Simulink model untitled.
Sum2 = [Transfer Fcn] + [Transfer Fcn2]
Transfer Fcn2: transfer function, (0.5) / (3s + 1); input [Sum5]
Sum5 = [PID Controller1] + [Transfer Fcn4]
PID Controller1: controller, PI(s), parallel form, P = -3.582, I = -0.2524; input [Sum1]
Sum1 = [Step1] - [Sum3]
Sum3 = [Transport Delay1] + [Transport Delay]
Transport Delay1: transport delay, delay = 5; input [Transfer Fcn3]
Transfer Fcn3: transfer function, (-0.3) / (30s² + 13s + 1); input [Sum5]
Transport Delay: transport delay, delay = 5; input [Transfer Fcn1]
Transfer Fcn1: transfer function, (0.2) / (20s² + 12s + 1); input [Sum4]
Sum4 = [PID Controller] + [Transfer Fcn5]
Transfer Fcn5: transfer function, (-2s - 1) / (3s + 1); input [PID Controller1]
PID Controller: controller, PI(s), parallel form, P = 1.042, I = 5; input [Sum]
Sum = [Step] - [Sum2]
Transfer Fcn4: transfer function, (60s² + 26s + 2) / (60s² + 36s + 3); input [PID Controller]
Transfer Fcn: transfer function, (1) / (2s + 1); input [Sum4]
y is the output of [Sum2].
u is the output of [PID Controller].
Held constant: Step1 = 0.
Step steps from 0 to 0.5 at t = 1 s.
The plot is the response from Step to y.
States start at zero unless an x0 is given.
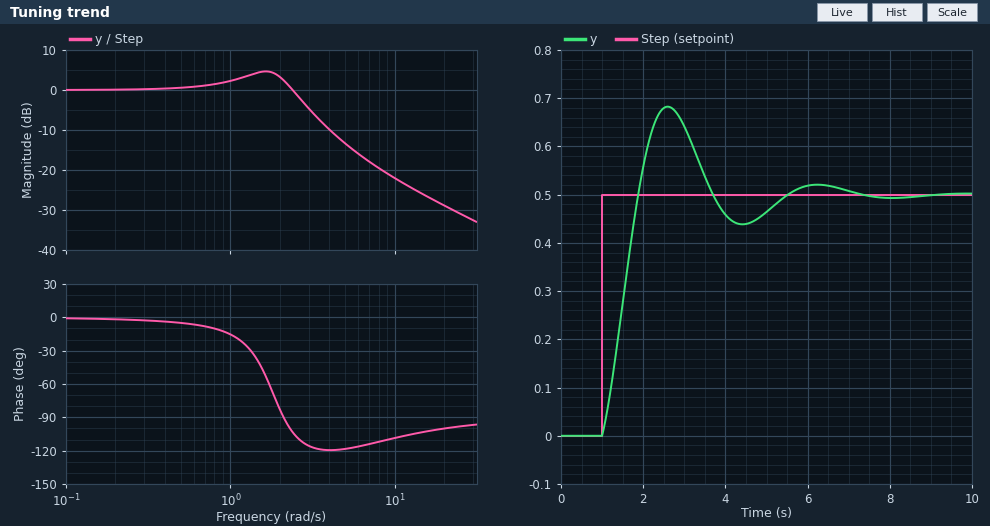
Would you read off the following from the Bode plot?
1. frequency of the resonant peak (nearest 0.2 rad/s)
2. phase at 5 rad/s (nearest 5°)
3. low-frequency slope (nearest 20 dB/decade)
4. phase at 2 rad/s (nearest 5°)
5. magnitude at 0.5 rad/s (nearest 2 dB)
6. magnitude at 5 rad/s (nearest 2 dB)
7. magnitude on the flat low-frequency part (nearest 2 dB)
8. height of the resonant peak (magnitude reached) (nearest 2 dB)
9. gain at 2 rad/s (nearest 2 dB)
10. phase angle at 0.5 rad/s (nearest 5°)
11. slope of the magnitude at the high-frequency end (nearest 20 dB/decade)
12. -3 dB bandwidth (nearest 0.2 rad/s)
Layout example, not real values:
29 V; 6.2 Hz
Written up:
1.6 rad/s; -120°; 0 dB/decade; -85°; 0 dB; -14 dB; 0 dB; 4 dB; 4 dB; -5°; -20 dB/decade; 2.8 rad/s
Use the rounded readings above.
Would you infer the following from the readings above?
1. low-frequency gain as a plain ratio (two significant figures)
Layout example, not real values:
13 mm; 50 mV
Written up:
1.0
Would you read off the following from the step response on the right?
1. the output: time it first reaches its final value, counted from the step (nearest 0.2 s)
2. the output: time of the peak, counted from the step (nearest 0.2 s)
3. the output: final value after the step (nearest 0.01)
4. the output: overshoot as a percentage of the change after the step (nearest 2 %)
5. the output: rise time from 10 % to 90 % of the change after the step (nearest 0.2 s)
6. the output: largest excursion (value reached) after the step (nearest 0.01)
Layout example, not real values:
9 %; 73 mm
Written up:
0.8 s; 1.6 s; 0.50; 36 %; 0.6 s; 0.68
